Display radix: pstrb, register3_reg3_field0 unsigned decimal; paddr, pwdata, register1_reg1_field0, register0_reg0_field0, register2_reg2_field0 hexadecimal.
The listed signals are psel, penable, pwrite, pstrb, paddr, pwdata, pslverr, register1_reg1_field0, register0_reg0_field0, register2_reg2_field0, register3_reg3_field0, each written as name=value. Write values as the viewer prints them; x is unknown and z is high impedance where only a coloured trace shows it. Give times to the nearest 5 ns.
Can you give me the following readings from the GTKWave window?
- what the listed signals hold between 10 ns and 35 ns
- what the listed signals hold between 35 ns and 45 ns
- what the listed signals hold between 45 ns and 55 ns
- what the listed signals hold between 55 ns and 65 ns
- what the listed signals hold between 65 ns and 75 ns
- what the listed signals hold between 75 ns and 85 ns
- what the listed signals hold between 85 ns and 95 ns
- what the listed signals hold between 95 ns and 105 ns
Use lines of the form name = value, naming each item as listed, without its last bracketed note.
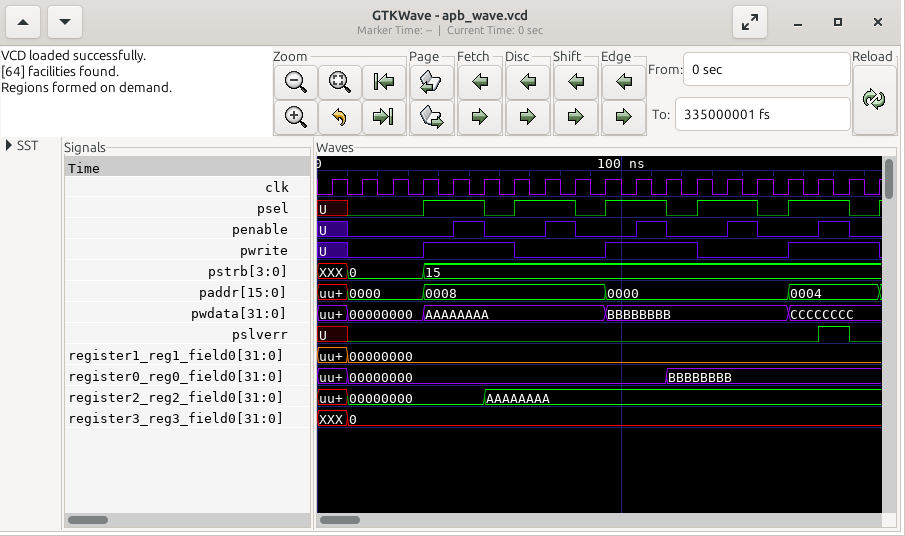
what the listed signals hold between 10 ns and 35 ns = psel=0, penable=0, pwrite=0, pstrb=0, paddr=0000, pwdata=00000000, pslverr=0, register1_reg1_field0=00000000, register0_reg0_field0=00000000, register2_reg2_field0=00000000, register3_reg3_field0=0
what the listed signals hold between 35 ns and 45 ns = psel=1, penable=0, pwrite=1, pstrb=15, paddr=0008, pwdata=AAAAAAAA, pslverr=0, register1_reg1_field0=00000000, register0_reg0_field0=00000000, register2_reg2_field0=00000000, register3_reg3_field0=0
what the listed signals hold between 45 ns and 55 ns = psel=1, penable=1, pwrite=1, pstrb=15, paddr=0008, pwdata=AAAAAAAA, pslverr=0, register1_reg1_field0=00000000, register0_reg0_field0=00000000, register2_reg2_field0=00000000, register3_reg3_field0=0
what the listed signals hold between 55 ns and 65 ns = psel=0, penable=0, pwrite=1, pstrb=15, paddr=0008, pwdata=AAAAAAAA, pslverr=0, register1_reg1_field0=00000000, register0_reg0_field0=00000000, register2_reg2_field0=AAAAAAAA, register3_reg3_field0=0
what the listed signals hold between 65 ns and 75 ns = psel=1, penable=0, pwrite=0, pstrb=15, paddr=0008, pwdata=AAAAAAAA, pslverr=0, register1_reg1_field0=00000000, register0_reg0_field0=00000000, register2_reg2_field0=AAAAAAAA, register3_reg3_field0=0
what the listed signals hold between 75 ns and 85 ns = psel=1, penable=1, pwrite=0, pstrb=15, paddr=0008, pwdata=AAAAAAAA, pslverr=0, register1_reg1_field0=00000000, register0_reg0_field0=00000000, register2_reg2_field0=AAAAAAAA, register3_reg3_field0=0
what the listed signals hold between 85 ns and 95 ns = psel=0, penable=0, pwrite=0, pstrb=15, paddr=0008, pwdata=AAAAAAAA, pslverr=0, register1_reg1_field0=00000000, register0_reg0_field0=00000000, register2_reg2_field0=AAAAAAAA, register3_reg3_field0=0
what the listed signals hold between 95 ns and 105 ns = psel=1, penable=0, pwrite=1, pstrb=15, paddr=0000, pwdata=BBBBBBBB, pslverr=0, register1_reg1_field0=00000000, register0_reg0_field0=00000000, register2_reg2_field0=AAAAAAAA, register3_reg3_field0=0
